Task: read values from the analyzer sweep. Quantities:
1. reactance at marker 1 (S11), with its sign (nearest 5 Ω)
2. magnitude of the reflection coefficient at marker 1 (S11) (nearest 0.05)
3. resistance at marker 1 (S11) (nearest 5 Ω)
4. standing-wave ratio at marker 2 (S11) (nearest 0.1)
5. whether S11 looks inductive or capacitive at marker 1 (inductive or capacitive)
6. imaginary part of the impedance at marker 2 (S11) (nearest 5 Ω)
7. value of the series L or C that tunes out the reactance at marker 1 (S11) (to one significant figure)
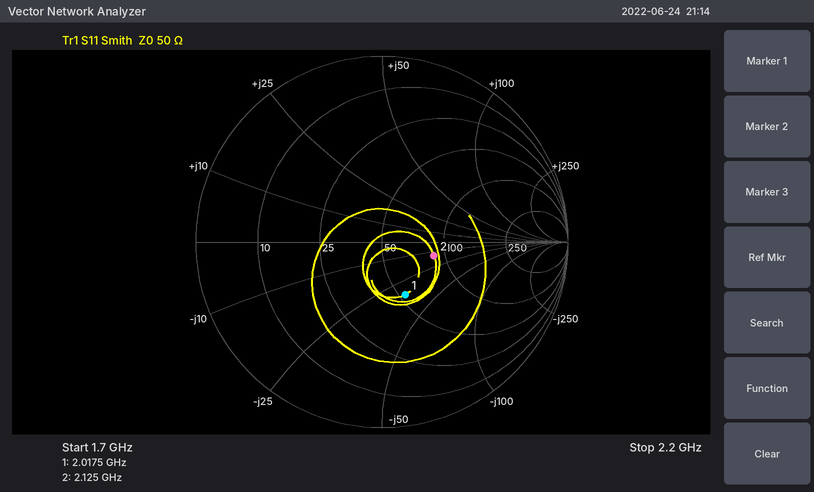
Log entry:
-35 Ω
0.30
55 Ω
1.8
capacitive
-15 Ω
3 nH
